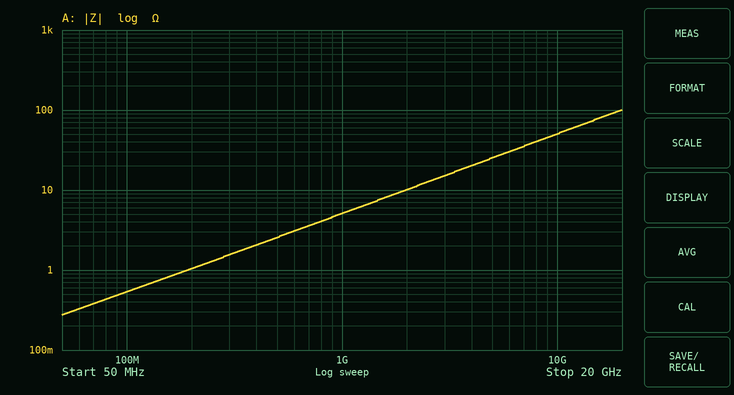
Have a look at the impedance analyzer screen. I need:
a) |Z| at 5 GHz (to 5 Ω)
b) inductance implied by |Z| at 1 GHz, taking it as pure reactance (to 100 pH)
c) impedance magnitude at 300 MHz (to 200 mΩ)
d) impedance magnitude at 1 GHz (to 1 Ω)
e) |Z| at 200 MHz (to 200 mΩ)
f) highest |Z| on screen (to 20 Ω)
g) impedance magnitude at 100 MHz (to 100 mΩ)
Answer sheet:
25 Ω
800 pH
1.6 Ω
5 Ω
1.0 Ω
100 Ω
500 mΩ
